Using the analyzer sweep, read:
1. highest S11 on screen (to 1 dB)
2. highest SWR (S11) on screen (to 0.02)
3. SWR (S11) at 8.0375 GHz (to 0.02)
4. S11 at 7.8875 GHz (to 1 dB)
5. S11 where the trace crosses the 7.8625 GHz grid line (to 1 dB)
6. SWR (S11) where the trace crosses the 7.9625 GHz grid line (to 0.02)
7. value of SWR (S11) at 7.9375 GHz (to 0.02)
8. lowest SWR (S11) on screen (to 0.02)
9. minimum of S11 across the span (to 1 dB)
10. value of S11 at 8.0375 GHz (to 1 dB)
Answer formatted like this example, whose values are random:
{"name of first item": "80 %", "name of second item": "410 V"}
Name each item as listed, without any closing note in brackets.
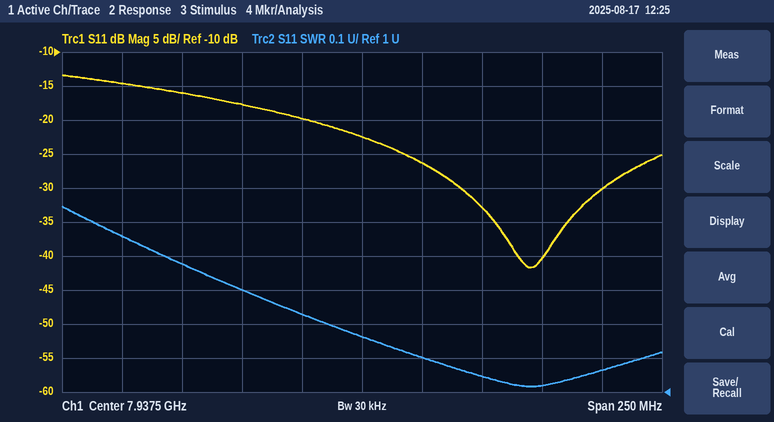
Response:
{"highest S11 on screen": "-13 dB", "highest SWR (S11) on screen": "1.54", "SWR (S11) at 8.0375 GHz": "1.06", "S11 at 7.8875 GHz": "-18 dB", "S11 where the trace crosses the 7.8625 GHz grid line": "-16 dB", "SWR (S11) where the trace crosses the 7.9625 GHz grid line": "1.10", "value of SWR (S11) at 7.9375 GHz": "1.16", "lowest SWR (S11) on screen": "1.02", "minimum of S11 across the span": "-42 dB", "value of S11 at 8.0375 GHz": "-30 dB"}
